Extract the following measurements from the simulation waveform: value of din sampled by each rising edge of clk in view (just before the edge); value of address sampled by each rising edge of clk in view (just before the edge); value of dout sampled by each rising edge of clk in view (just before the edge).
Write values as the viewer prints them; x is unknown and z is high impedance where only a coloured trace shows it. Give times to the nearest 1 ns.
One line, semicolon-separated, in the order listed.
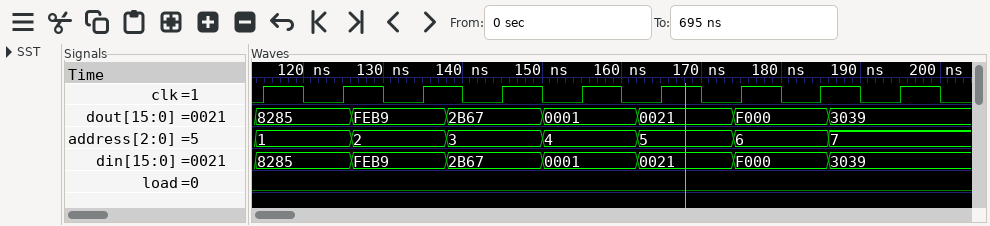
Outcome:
8285, 8285, FEB9, 2B67, 0001, 0021, F000, F000, 3039; 1, 1, 2, 3, 4, 5, 6, 6, 7; 8285, 8285, FEB9, 2B67, 0001, 0021, F000, F000, 3039
